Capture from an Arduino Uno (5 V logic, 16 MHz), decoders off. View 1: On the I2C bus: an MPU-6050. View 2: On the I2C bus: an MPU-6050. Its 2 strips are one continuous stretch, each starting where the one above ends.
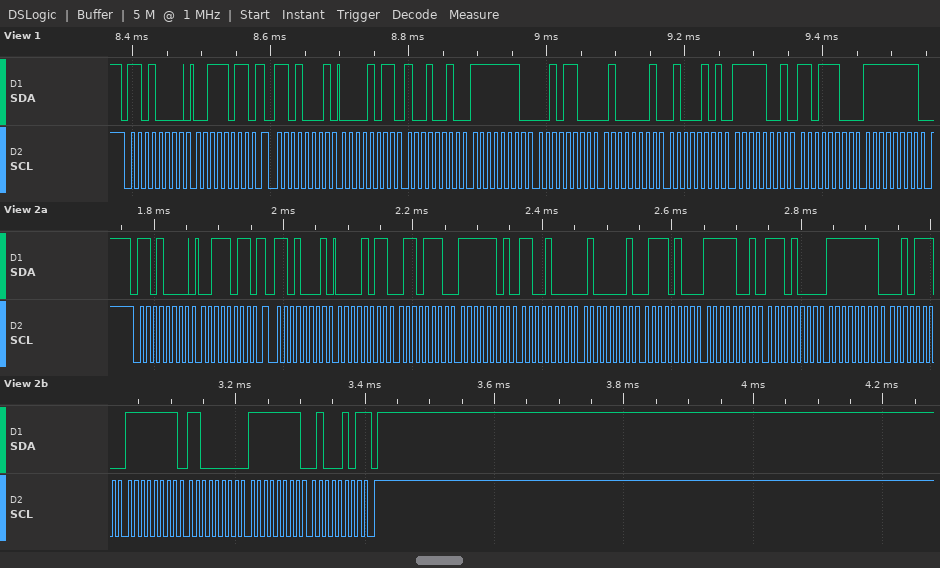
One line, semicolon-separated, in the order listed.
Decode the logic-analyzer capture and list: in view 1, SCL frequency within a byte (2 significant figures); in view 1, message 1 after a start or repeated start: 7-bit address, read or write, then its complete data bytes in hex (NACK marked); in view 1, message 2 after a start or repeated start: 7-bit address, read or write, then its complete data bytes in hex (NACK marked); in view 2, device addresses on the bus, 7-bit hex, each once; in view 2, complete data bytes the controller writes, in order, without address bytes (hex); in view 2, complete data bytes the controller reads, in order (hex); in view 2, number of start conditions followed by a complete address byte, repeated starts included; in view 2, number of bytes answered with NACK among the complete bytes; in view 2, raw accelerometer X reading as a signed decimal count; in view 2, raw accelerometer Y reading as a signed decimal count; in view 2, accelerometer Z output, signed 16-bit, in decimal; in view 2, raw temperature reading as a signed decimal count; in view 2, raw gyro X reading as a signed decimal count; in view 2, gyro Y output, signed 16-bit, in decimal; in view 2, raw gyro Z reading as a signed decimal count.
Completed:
100 kHz; 0x68 write: 3B; 0x68 read: 0B 92 FE 2C 41 45 F9 DC FF; 0x68; 3B; 0B 6E FD C8 41 74 F9 E8 FF 2E FF C0 FF 45; 2; 1; 2926; -568; 16756; -1560; -210; -64; -187
